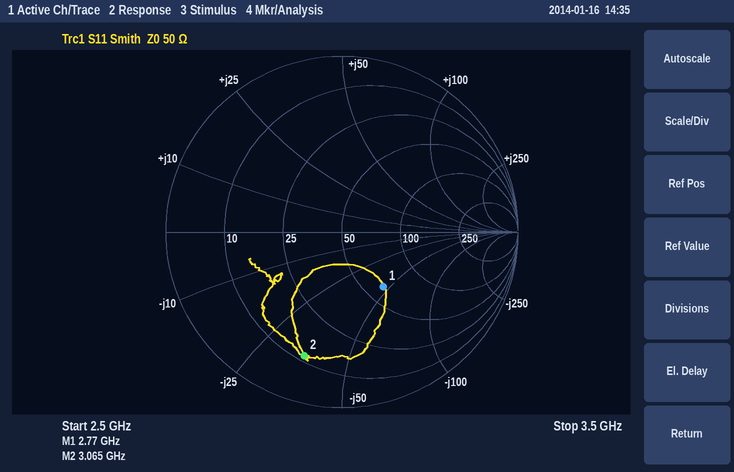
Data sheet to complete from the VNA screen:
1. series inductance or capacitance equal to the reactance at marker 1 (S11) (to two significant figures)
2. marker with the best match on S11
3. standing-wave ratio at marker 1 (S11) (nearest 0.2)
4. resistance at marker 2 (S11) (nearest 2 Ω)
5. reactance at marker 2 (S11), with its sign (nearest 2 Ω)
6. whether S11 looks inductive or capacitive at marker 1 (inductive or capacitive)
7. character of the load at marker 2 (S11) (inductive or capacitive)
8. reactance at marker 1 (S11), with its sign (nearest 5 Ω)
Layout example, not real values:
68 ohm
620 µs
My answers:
1.3 pF
marker 1
2.2
12 Ω
-36 Ω
capacitive
capacitive
-45 Ω
